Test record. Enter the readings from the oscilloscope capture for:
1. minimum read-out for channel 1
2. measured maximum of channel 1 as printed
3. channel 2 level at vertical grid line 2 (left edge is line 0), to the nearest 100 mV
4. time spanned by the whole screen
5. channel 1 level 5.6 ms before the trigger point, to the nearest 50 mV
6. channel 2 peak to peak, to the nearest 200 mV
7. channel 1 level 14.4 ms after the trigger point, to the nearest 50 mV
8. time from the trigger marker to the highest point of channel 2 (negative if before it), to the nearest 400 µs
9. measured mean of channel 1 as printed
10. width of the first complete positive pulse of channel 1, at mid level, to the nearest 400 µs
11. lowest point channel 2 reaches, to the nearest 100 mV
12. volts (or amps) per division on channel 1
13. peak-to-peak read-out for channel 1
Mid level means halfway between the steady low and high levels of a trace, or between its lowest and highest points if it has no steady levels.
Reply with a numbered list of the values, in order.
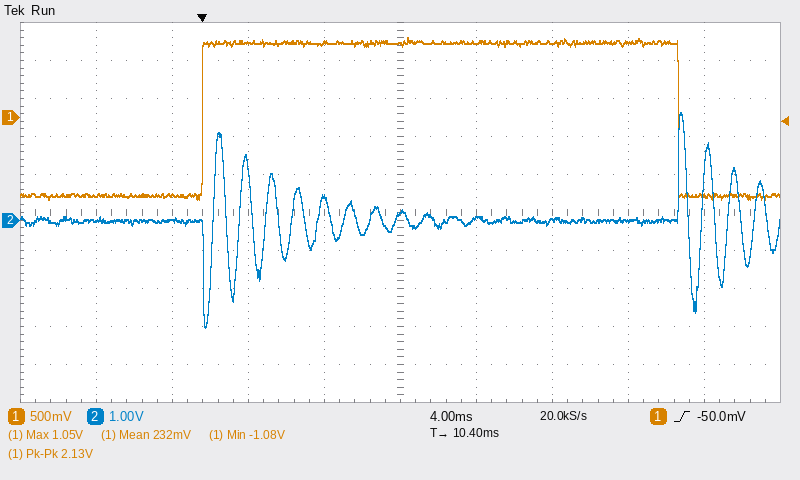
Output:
1. -1.08 V
2. 1.05 V
3. 0.0 V
4. 40 ms
5. -1.00 V
6. 5.6 V
7. 1.00 V
8. +25.2 ms
9. 232 mV
10. 25.2 ms
11. -2.8 V
12. 500 mV
13. 2.13 V
